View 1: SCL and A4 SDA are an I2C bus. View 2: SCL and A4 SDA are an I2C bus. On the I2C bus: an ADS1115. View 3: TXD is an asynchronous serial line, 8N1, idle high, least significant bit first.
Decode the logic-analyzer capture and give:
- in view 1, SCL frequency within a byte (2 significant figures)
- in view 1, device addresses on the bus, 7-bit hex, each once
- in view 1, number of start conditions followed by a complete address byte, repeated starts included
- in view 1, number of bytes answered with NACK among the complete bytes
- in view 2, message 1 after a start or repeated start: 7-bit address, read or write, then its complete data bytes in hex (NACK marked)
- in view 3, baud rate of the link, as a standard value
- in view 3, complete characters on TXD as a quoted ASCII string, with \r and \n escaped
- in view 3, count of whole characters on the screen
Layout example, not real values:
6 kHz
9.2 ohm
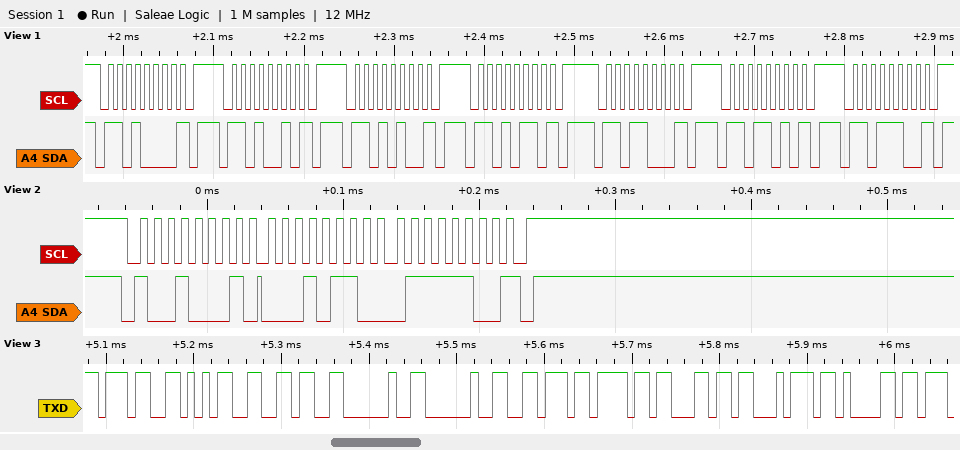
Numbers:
100 kHz
0x68 0x69 0x6A 0x6B 0x6C 0x6D 0x6E
7
7
0x48 read: 16 7C NACK
115200 baud
"756  volta"
10
